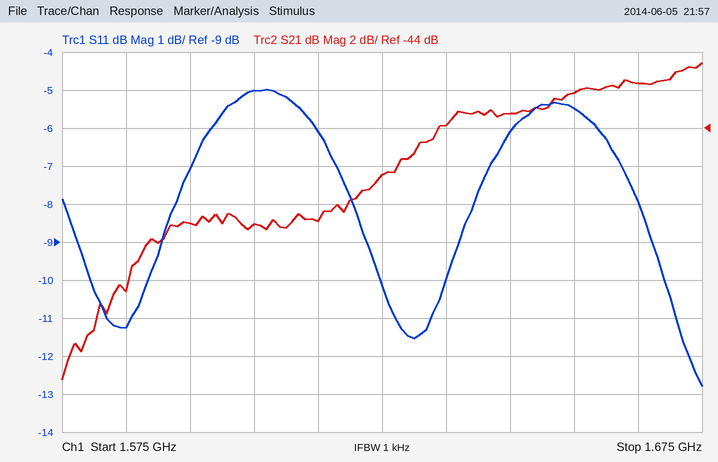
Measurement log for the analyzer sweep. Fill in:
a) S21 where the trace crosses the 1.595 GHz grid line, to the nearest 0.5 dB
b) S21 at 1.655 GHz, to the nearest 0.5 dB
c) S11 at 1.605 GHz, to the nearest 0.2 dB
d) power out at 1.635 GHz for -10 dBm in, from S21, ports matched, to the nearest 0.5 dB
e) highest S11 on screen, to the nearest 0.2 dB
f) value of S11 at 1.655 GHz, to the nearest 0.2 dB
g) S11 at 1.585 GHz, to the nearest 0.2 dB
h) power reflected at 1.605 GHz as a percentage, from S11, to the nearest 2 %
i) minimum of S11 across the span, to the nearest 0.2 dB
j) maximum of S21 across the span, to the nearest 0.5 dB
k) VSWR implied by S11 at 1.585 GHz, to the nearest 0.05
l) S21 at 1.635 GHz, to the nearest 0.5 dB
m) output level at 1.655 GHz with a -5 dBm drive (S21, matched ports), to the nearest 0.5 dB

-49.0 dB
-42.0 dB
-5.0 dB
-54.0 dBm
-5.0 dB
-5.4 dB
-11.2 dB
32 %
-12.8 dB
-40.5 dB
1.75
-44.0 dB
-47.0 dBm
